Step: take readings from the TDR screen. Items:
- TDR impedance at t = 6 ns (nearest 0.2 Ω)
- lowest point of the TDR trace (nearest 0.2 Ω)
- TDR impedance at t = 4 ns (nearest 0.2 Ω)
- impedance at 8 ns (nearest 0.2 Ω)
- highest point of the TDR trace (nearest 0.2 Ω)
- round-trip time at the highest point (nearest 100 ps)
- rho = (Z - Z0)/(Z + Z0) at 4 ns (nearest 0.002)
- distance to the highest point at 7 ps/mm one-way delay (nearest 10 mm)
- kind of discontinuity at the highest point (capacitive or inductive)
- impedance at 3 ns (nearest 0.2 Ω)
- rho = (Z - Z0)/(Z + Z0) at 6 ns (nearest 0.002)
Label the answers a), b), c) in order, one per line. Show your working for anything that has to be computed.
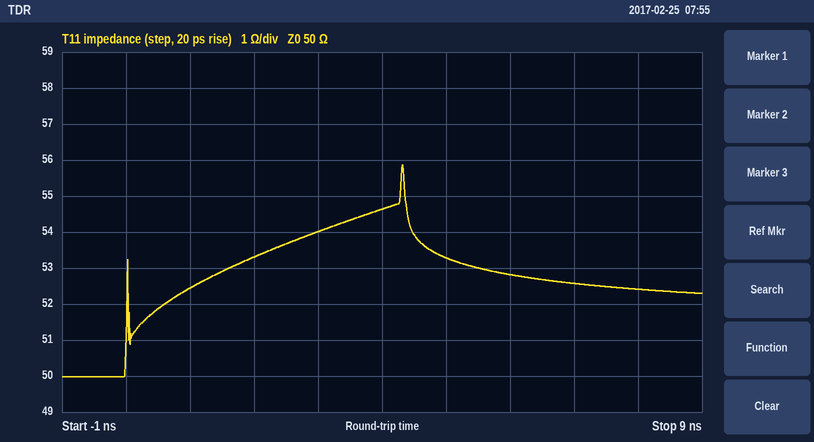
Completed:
a) 52.8 Ω
b) 50.0 Ω
c) 54.6 Ω
d) 52.4 Ω
e) 55.8 Ω
f) 4.3 ns
g) (54.6 − 50)/(54.6 + 50) ≈ +0.044
h) 4.3 ns / 2 / 7 ps/mm ≈ 307 mm, so 310 mm to the nearest 10 mm
i) inductive
j) 54.0 Ω
k) (52.8 − 50)/(52.8 + 50) ≈ +0.0272, so +0.028 to the nearest 0.002
